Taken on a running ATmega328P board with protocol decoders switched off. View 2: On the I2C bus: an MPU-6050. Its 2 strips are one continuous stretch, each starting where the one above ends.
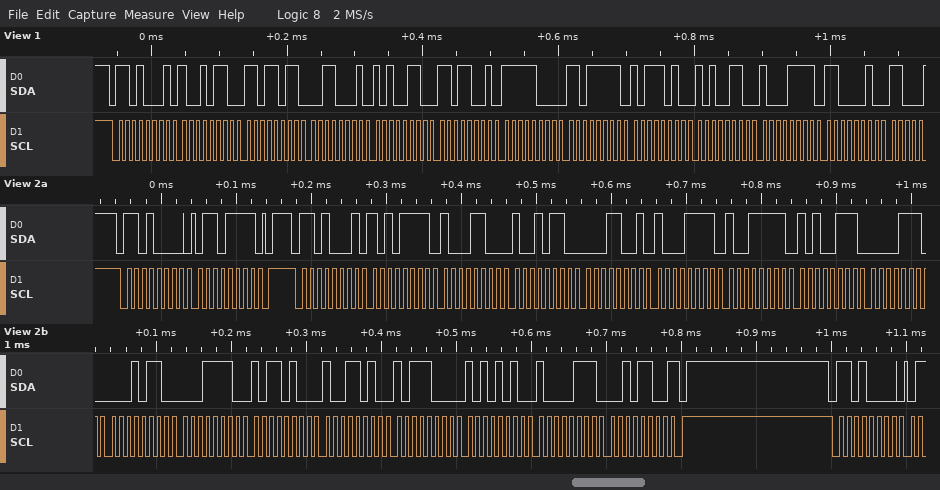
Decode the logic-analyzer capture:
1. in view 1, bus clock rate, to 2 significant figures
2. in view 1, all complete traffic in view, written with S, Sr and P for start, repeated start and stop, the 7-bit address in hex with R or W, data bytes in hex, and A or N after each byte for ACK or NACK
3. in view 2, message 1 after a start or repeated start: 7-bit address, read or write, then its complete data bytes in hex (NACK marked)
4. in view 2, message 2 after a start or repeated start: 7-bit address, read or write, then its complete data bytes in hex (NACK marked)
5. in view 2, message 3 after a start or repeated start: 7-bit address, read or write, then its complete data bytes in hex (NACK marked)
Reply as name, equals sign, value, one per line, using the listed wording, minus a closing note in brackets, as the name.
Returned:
in view 1, bus clock rate, to 2 significant figures = 100 kHz
in view 1, all complete traffic in view, written with S, Sr and P for start, repeated start and stop, the 7-bit address in hex with R or W, data bytes in hex, and A or N after each byte for ACK or NACK = S 68R A 96 A DB A 31 A A6 A D9 A F8 A DF A BA A A6 A 8F A C2 A
in view 2, message 1 after a start or repeated start: 7-bit address, read or write, then its complete data bytes in hex = 0x68 write: 6F
in view 2, message 2 after a start or repeated start: 7-bit address, read or write, then its complete data bytes in hex = 0x68 read: AF 8C 96 19 8F 9F A7 0E 16 1E B4 9A B8 AA 87 2C NACK
in view 2, message 3 after a start or repeated start: 7-bit address, read or write, then its complete data bytes in hex = 0x68 write
